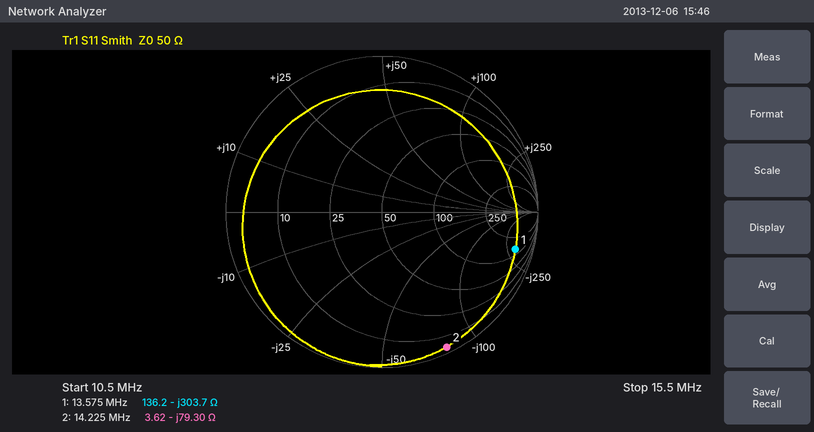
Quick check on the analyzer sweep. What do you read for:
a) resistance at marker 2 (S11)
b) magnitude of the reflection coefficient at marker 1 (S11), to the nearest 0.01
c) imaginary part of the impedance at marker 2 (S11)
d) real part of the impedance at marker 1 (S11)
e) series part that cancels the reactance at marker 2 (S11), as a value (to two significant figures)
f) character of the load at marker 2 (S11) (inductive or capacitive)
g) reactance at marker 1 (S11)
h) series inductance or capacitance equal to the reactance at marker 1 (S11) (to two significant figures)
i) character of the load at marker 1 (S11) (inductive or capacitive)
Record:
3.62 Ω
0.89
-79.30 Ω
136.2 Ω
890 nH
capacitive
-303.7 Ω
39 pF
capacitive
